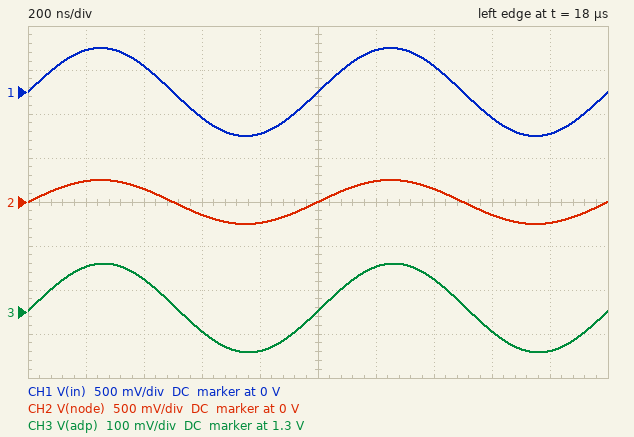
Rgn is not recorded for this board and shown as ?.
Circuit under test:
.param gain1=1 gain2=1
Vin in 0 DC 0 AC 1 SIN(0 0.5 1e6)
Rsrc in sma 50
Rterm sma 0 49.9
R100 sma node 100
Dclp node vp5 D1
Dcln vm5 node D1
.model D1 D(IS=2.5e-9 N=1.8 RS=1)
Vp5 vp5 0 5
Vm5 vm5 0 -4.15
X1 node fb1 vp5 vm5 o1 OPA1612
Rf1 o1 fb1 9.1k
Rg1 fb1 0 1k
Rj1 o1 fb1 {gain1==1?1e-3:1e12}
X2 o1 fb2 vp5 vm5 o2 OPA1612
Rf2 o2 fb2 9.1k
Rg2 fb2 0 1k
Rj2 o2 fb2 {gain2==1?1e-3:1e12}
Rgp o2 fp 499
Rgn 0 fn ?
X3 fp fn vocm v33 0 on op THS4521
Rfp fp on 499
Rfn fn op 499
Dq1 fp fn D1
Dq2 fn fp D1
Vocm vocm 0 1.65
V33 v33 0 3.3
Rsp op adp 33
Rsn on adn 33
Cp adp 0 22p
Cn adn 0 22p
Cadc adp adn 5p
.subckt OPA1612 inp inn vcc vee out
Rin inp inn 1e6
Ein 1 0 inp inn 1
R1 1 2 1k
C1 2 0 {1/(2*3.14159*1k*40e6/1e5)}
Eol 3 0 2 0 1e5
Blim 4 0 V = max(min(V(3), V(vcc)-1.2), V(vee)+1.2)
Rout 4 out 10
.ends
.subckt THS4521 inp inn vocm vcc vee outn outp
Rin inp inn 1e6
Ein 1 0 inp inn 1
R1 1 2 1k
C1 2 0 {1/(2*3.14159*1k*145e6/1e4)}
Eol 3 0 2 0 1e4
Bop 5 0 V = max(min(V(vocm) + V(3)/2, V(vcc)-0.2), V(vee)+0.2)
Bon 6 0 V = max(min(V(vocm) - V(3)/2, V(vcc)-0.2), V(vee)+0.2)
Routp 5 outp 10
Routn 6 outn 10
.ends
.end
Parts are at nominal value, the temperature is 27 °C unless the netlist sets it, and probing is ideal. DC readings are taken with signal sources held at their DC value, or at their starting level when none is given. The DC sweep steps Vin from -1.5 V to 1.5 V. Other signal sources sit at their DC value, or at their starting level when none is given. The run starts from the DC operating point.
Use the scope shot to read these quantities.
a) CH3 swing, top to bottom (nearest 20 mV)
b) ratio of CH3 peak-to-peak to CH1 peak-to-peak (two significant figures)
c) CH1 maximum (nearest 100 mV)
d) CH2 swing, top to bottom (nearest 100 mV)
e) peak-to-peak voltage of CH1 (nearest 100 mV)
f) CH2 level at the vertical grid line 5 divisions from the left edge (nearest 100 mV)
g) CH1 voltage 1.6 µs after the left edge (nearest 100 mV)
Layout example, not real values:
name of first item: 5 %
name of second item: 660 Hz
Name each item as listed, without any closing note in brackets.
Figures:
CH3 swing, top to bottom: 200 mV
ratio of CH3 peak-to-peak to CH1 peak-to-peak: 0.20
CH1 maximum: 500 mV
CH2 swing, top to bottom: 500 mV
peak-to-peak voltage of CH1: 1.0 V
CH2 level at the vertical grid line 5 divisions from the left edge: 0 V
CH1 voltage 1.6 µs after the left edge: -300 mV
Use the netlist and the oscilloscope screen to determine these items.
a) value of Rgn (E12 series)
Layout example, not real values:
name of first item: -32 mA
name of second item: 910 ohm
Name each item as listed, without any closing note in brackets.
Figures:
value of Rgn: 1.5 kΩ
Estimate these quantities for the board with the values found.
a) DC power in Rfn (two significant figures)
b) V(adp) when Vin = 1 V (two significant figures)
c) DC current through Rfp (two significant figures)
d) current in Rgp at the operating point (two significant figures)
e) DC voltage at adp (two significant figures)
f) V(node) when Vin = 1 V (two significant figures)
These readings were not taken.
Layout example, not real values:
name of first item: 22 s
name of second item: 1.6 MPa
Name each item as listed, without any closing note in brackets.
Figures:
DC power in Rfn: 210 µW
V(adp) when Vin = 1 V: 1.5 V
DC current through Rfp: 2.0 mA
current in Rgp at the operating point: 2.0 mA
DC voltage at adp: 1.3 V
V(node) when Vin = 1 V: 500 mV
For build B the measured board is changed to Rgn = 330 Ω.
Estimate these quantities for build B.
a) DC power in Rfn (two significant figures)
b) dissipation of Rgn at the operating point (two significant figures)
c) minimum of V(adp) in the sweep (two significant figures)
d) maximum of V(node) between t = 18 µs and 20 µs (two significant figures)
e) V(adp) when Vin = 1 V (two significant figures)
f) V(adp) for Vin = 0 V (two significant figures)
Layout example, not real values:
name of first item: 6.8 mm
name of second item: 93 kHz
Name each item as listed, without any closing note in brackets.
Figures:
DC power in Rfn: 2.4 mW
dissipation of Rgn at the operating point: 1.6 mW
minimum of V(adp) in the sweep: 1.4 V
maximum of V(node) between t = 18 µs and 20 µs: 250 mV
V(adp) when Vin = 1 V: 2.1 V
V(adp) for Vin = 0 V: 1.8 V
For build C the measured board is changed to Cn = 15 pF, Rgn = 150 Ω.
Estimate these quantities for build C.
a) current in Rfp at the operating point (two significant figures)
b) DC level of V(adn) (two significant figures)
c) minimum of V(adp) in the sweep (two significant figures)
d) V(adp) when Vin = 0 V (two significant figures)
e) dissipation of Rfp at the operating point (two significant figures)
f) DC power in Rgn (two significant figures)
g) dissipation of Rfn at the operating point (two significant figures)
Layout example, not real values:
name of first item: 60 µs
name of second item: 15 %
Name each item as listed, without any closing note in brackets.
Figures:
current in Rfp at the operating point: 1.0 mA
DC level of V(adn): 1.0 V
minimum of V(adp) in the sweep: 1.7 V
V(adp) when Vin = 0 V: 2.2 V
dissipation of Rfp at the operating point: 530 µW
DC power in Rgn: 1.8 mW
dissipation of Rfn at the operating point: 5.9 mW
